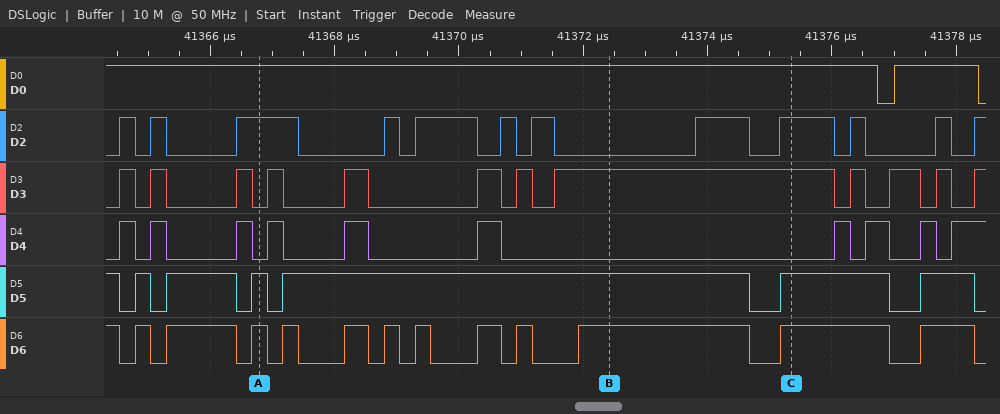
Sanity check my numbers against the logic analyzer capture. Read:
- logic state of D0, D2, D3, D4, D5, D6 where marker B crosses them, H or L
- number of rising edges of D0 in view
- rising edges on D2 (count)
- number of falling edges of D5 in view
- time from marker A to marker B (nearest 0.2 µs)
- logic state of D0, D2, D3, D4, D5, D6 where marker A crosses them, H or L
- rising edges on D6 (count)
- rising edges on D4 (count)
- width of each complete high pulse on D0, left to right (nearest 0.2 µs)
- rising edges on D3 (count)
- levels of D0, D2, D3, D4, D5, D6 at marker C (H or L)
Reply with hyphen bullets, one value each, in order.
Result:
- D0=H, D2=L, D3=H, D4=L, D5=H, D6=H
- 1
- 12
- 7
- 5.6 µs
- D0=H, D2=H, D3=L, D4=L, D5=H, D6=H
- 12
- 10
- 1.4 µs
- 12
- D0=H, D2=H, D3=H, D4=L, D5=H, D6=H
